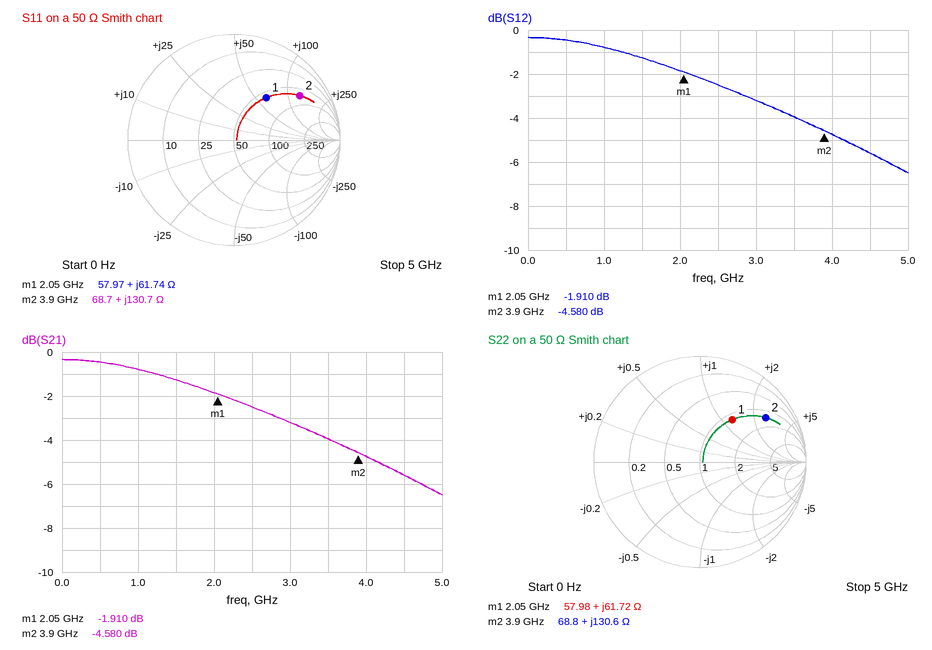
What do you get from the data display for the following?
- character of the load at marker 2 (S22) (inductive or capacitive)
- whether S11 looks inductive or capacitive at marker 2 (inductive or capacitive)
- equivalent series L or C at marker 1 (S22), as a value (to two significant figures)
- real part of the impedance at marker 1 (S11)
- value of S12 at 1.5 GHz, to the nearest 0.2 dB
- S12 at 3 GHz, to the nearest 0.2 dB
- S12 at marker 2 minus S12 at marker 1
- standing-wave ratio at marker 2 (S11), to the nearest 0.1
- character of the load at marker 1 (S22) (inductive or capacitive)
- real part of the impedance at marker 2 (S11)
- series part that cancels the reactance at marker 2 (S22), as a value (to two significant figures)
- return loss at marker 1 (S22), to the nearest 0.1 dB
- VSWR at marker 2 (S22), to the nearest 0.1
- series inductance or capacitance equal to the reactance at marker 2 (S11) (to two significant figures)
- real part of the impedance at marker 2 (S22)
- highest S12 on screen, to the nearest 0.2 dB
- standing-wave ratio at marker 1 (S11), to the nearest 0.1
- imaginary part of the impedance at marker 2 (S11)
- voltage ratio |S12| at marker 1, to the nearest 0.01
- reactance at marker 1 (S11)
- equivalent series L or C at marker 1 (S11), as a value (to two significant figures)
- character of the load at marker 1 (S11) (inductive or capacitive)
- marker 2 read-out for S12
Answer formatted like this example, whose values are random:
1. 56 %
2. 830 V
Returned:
1. inductive
2. inductive
3. 4.8 nH
4. 57.97 Ω
5. -1.2 dB
6. -3.2 dB
7. -2.670 dB
8. 6.9
9. inductive
10. 68.7 Ω
11. 310 fF
12. 6.0 dB
13. 6.9
14. 5.3 nH
15. 68.8 Ω
16. -0.4 dB
17. 3.0
18. +130.7 Ω
19. 0.80
20. +61.74 Ω
21. 4.8 nH
22. inductive
23. -4.580 dB
